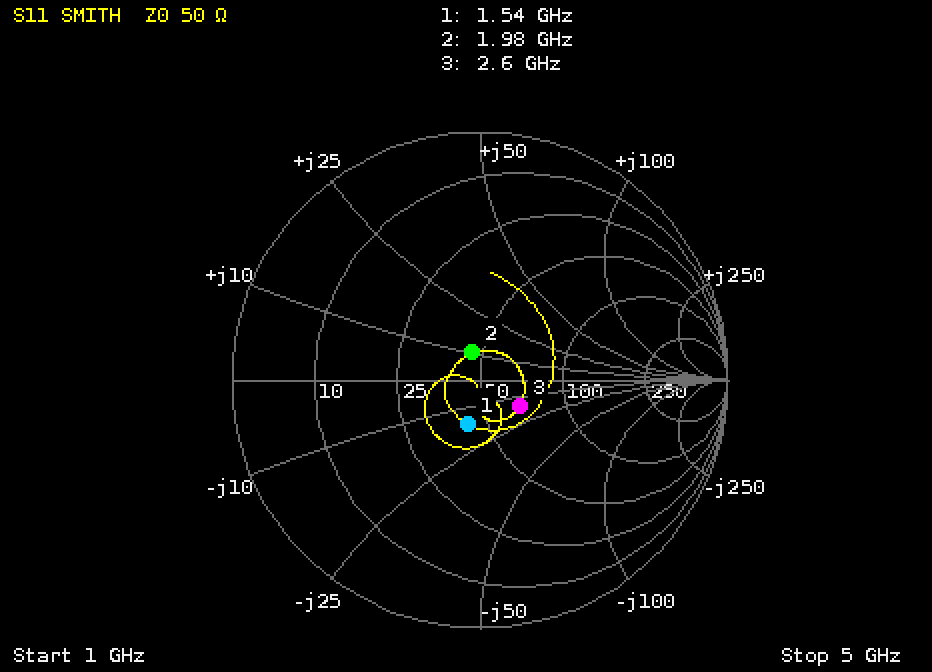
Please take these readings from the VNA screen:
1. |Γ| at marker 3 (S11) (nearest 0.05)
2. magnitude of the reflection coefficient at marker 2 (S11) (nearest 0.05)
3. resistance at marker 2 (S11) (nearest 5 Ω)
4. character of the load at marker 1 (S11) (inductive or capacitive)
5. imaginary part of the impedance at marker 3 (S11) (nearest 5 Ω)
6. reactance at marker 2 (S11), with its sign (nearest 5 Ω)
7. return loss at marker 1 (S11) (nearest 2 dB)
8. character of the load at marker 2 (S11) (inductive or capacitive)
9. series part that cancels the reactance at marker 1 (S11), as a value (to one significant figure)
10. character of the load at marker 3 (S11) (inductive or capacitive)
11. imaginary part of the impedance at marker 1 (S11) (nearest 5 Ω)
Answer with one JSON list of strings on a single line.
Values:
["0.20", "0.10", "45 Ω", "capacitive", "-15 Ω", "+10 Ω", "14 dB", "inductive", "2 nH", "capacitive", "-15 Ω"]
